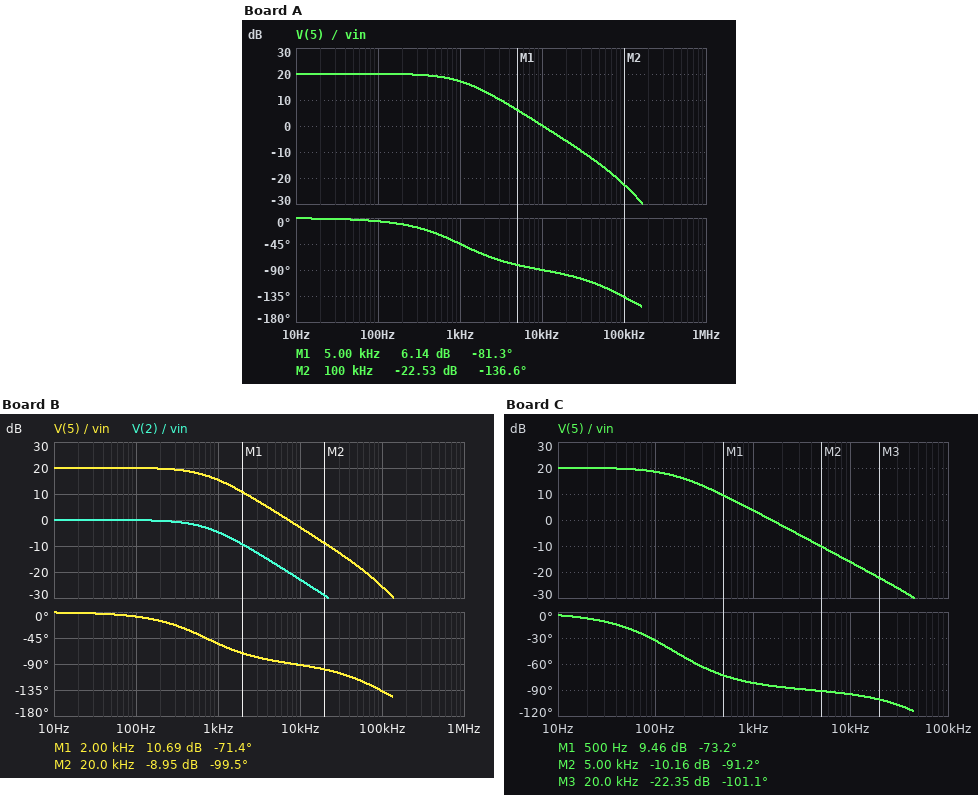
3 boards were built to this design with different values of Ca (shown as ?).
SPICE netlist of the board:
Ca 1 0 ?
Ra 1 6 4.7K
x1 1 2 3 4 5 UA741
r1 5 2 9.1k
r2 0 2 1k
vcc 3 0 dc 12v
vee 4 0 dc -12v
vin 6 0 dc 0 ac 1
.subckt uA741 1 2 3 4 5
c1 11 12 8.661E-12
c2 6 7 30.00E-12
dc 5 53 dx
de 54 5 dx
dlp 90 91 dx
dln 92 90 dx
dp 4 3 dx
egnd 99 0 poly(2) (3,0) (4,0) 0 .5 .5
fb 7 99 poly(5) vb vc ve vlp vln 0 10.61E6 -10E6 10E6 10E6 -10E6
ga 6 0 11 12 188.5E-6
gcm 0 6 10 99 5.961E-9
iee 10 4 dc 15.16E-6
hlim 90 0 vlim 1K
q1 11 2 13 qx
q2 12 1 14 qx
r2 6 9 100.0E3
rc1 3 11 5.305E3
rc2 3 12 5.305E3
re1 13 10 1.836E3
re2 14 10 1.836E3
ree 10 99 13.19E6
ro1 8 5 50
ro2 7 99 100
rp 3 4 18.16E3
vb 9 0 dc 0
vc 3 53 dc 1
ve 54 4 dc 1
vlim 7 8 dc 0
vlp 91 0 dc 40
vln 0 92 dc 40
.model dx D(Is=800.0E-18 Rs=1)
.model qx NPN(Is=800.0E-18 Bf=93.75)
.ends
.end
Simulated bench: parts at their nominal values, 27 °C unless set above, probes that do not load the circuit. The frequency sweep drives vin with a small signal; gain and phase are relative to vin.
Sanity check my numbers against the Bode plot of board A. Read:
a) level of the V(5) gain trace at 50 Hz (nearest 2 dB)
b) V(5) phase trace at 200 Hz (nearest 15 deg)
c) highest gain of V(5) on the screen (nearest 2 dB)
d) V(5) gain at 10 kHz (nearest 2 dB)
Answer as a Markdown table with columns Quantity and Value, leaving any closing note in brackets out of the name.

| Quantity | Value |
|---|---|
| level of the V(5) gain trace at 50 Hz | 20 dB |
| V(5) phase trace at 200 Hz | -15 deg |
| highest gain of V(5) on the screen | 20 dB |
| V(5) gain at 10 kHz | 0 dB |
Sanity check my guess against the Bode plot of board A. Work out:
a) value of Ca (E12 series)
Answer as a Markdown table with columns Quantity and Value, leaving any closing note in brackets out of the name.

| Quantity | Value |
|---|---|
| value of Ca | 33 nF |
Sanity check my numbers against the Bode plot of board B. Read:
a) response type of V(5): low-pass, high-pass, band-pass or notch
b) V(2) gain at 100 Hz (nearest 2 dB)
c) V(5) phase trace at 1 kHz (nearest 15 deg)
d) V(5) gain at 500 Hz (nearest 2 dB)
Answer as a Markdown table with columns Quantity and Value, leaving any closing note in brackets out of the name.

| Quantity | Value |
|---|---|
| response type of V(5): low-pass, high-pass, band-pass or notch | low-pass |
| V(2) gain at 100 Hz | 0 dB |
| V(5) phase trace at 1 kHz | -60 deg |
| V(5) gain at 500 Hz | 18 dB |
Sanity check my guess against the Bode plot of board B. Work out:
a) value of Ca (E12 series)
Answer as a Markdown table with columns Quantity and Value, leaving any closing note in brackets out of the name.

| Quantity | Value |
|---|---|
| value of Ca | 47 nF |
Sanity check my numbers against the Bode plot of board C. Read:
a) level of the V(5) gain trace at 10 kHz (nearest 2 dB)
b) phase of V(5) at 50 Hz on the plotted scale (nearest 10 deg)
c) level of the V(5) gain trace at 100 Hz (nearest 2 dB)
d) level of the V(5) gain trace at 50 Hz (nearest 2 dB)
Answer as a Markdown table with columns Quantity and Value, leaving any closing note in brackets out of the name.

| Quantity | Value |
|---|---|
| level of the V(5) gain trace at 10 kHz | -16 dB |
| phase of V(5) at 50 Hz on the plotted scale | -20 deg |
| level of the V(5) gain trace at 100 Hz | 18 dB |
| level of the V(5) gain trace at 50 Hz | 20 dB |
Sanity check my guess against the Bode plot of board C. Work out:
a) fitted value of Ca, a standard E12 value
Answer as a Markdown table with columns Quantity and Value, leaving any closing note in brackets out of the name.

| Quantity | Value |
|---|---|
| fitted value of Ca, a standard E12 value | 220 nF |
